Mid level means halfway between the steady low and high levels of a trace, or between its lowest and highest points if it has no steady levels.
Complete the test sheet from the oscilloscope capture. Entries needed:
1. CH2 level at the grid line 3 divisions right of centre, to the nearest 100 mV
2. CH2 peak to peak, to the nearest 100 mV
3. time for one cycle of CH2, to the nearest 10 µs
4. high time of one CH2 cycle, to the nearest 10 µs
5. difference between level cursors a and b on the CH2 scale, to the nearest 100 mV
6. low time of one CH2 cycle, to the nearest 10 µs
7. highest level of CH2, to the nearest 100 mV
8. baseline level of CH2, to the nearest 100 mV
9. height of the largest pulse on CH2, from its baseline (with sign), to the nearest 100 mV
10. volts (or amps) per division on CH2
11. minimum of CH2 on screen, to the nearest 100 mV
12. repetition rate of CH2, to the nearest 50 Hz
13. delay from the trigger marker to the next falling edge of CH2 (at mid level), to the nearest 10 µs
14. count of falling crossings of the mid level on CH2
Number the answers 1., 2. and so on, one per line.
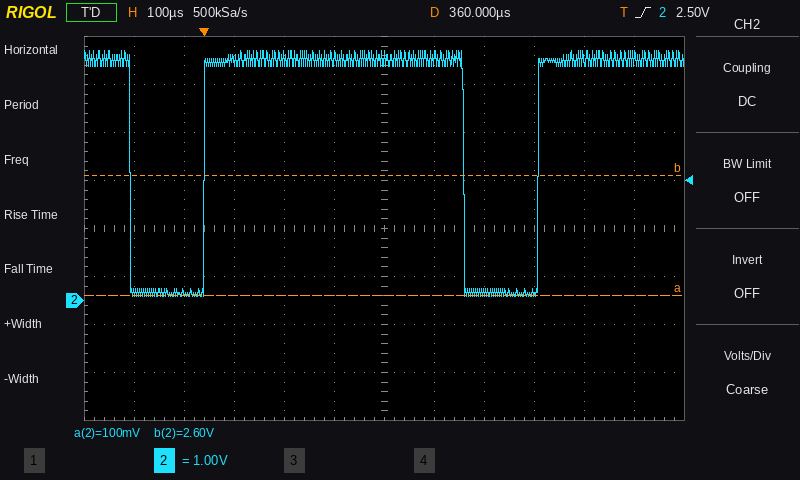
1. 200 mV
2. 5.1 V
3. 670 µs
4. 520 µs
5. 2.5 V
6. 150 µs
7. 5.2 V
8. 5.0 V
9. -4.9 V
10. 1 V
11. 100 mV
12. 1.50 kHz
13. 520 µs
14. 2
